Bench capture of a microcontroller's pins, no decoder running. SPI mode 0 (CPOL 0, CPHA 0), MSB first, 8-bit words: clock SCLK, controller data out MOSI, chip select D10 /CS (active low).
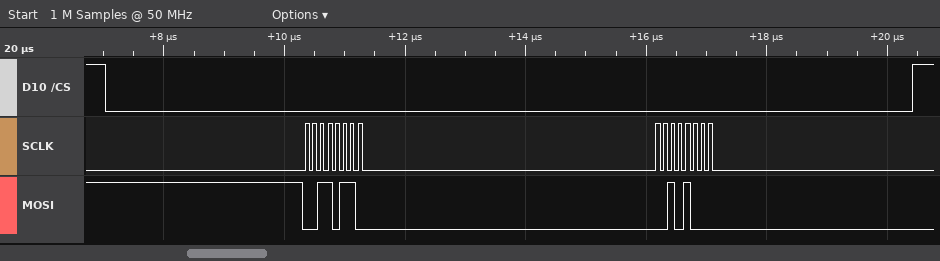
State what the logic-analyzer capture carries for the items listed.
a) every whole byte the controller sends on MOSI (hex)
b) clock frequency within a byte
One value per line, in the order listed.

0x36 0x28
8 MHz
